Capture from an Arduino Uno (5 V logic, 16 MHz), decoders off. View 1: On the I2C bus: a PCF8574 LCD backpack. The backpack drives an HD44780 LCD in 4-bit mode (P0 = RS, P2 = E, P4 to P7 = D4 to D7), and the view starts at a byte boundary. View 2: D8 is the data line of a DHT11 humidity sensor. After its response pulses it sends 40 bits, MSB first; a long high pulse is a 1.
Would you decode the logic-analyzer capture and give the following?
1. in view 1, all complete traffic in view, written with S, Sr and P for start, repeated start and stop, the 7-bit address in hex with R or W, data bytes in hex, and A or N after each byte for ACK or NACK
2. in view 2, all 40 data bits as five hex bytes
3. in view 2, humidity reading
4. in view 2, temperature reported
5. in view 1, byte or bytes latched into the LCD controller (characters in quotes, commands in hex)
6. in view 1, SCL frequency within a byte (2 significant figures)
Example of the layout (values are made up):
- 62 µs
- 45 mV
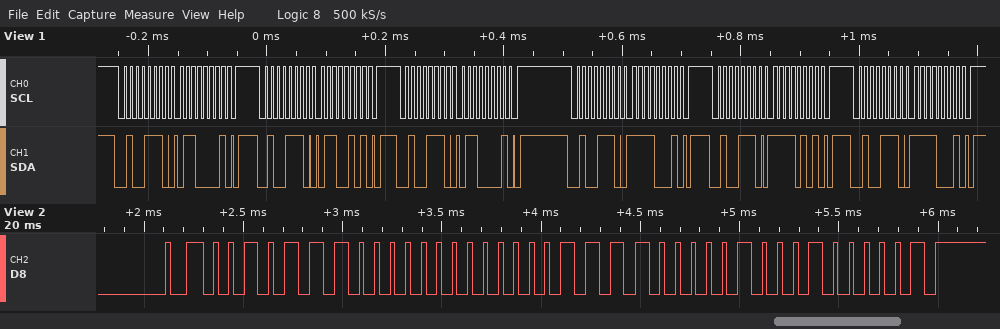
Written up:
- S 27W A 61 A P S 27W A 65 A P S 27W A 61 A P S 27W A F1 A P S 27W A F5 A P S 27W A F1 A P
- 2E 00 0F 04 41
- 46 %
- 15.4 °C
- 'o'
- 100 kHz
